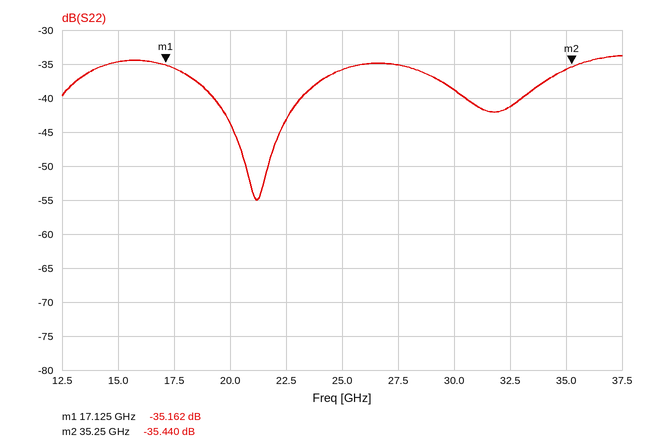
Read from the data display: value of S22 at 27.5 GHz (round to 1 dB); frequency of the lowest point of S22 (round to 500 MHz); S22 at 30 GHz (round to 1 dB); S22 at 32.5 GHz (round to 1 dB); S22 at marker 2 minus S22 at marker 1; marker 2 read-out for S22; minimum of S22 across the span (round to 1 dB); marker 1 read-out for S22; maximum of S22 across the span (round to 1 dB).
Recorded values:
-35 dB
21.0 GHz
-39 dB
-41 dB
-0.278 dB
-35.440 dB
-55 dB
-35.162 dB
-34 dB
